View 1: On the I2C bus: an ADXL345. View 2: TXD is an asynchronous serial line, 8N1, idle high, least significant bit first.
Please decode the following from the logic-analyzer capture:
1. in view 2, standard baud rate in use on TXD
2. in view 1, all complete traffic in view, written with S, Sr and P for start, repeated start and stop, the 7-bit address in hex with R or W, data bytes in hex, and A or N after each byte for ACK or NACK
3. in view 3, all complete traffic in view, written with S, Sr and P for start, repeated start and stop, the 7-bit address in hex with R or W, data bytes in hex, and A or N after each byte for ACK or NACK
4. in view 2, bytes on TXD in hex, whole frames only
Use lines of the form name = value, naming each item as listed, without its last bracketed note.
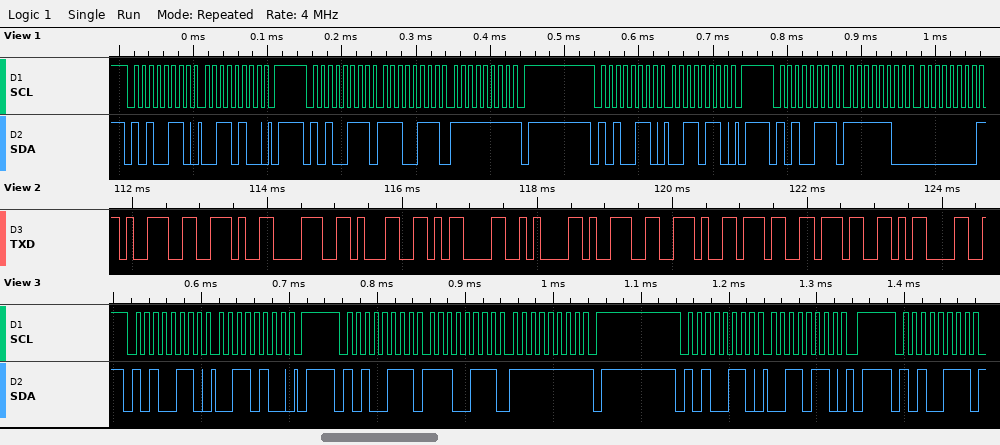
in view 2, standard baud rate in use on TXD = 9600 baud
in view 1, all complete traffic in view, written with S, Sr and P for start, repeated start and stop, the 7-bit address in hex with R or W, data bytes in hex, and A or N after each byte for ACK or NACK = S 53W A 34 A P S 53R A E7 A FF N P S 53W A 36 A P S 53R A FC A 00 N
in view 3, all complete traffic in view, written with S, Sr and P for start, repeated start and stop, the 7-bit address in hex with R or W, data bytes in hex, and A or N after each byte for ACK or NACK = S 53W A 34 A P S 53R A E7 A FF N P S 53W A 36 A P S 53R A
in view 2, bytes on TXD in hex, whole frames only = 39 2E 38 31 0D 0A 39 2E 37 37 0D
